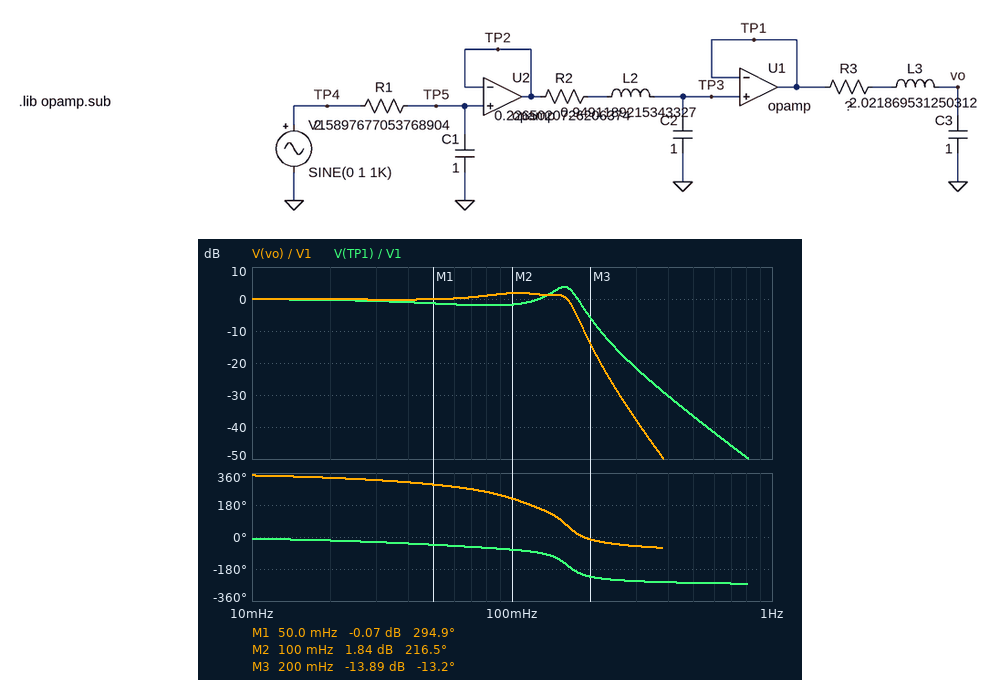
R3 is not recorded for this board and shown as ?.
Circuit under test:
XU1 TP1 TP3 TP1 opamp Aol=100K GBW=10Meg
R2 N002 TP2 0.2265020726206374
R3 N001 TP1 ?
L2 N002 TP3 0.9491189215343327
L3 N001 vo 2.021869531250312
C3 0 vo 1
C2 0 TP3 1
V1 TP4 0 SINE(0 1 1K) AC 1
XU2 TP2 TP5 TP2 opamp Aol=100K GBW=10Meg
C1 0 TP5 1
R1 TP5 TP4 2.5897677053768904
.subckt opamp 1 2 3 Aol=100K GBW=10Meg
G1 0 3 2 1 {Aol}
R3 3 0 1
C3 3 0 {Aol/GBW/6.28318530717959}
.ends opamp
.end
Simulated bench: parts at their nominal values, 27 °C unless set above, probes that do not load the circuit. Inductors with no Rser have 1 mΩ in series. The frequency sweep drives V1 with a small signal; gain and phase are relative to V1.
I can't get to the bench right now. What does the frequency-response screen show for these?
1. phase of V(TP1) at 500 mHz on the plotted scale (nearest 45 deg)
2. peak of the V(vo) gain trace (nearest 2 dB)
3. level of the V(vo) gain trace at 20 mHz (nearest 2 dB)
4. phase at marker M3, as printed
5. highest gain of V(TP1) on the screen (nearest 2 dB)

-270 deg
2 dB
0 dB
-13.2 deg
4 dB
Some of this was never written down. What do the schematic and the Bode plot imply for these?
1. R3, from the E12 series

1 Ω
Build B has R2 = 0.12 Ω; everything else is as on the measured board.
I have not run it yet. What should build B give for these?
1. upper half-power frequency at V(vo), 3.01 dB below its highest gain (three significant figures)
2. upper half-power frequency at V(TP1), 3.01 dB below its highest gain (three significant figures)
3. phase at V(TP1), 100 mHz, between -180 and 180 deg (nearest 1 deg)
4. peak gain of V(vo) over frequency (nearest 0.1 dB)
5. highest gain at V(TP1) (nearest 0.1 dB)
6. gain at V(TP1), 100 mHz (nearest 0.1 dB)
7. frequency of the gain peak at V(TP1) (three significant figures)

169 mHz
172 mHz
-65 deg
5.7 dB
9.1 dB
-1.6 dB
162 mHz
